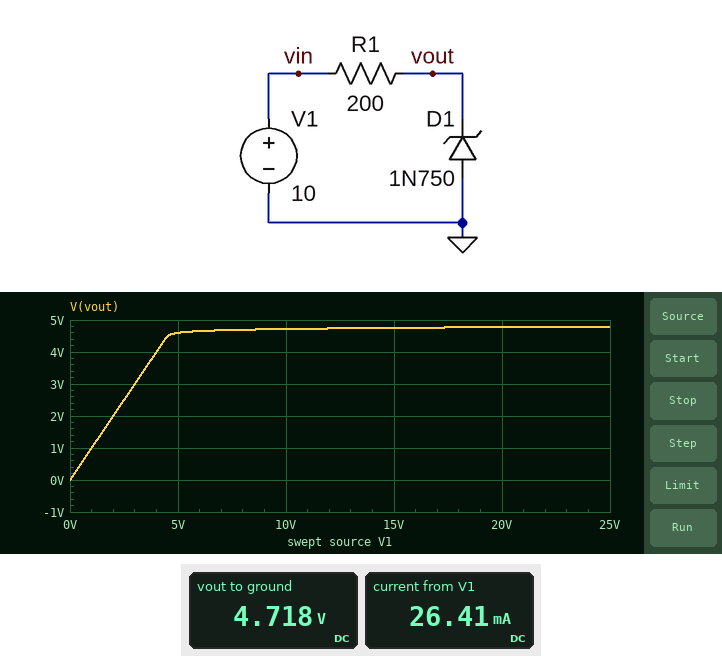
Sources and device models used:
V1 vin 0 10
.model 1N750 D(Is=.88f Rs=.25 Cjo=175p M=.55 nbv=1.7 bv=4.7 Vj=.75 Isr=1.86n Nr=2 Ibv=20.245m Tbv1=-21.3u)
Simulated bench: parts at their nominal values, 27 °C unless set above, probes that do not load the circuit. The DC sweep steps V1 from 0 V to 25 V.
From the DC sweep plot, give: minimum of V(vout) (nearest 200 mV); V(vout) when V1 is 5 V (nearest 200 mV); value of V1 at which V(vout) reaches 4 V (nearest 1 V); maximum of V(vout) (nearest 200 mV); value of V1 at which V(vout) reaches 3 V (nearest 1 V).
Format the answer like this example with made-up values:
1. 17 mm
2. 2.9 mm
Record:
1. 0 V
2. 4.6 V
3. 4 V
4. 4.8 V
5. 3 V
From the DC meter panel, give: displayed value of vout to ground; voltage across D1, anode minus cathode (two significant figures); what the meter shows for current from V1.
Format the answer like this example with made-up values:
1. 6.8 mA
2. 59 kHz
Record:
1. 4.718 V
2. -4.7 V
3. 26.41 mA
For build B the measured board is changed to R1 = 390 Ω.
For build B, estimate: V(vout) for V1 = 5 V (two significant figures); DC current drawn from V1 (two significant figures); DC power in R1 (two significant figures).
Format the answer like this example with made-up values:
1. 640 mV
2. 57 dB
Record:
1. 4.6 V
2. 14 mA
3. 72 mW
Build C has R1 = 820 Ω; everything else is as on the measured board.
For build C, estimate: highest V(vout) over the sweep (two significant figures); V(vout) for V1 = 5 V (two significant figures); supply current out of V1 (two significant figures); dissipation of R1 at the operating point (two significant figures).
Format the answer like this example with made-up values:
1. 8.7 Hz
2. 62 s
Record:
1. 4.7 V
2. 4.5 V
3. 6.5 mA
4. 35 mW
